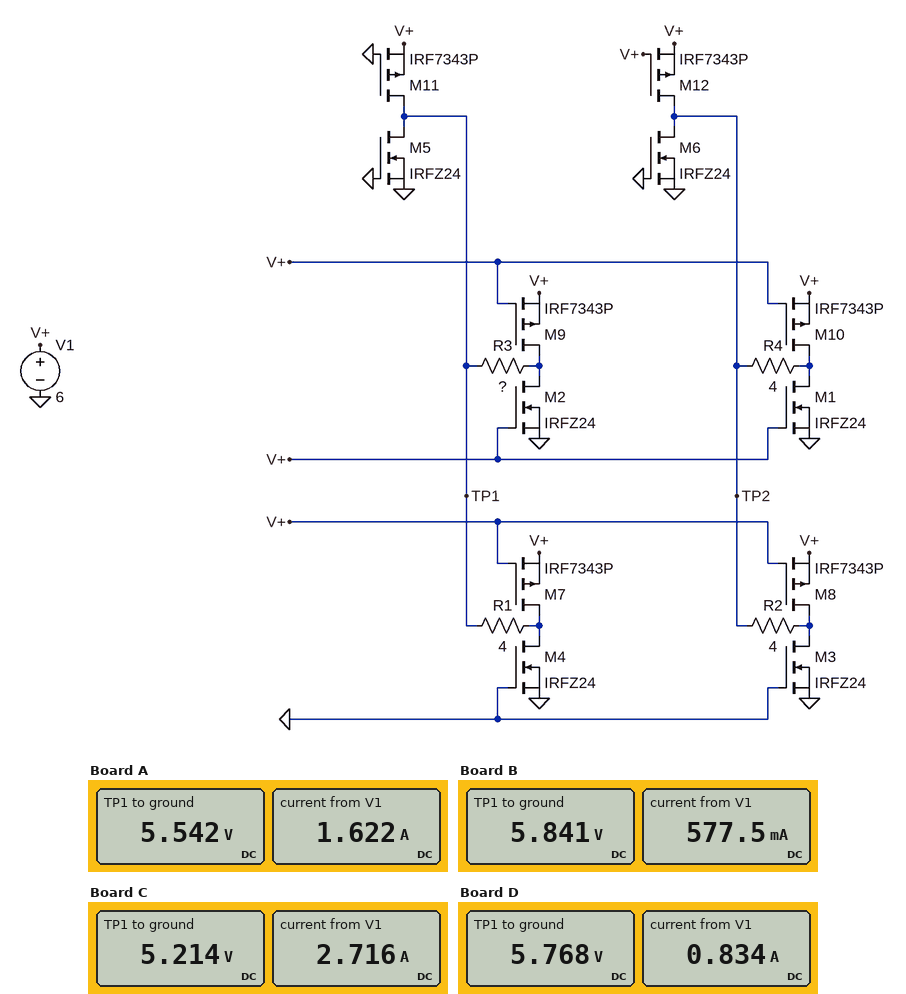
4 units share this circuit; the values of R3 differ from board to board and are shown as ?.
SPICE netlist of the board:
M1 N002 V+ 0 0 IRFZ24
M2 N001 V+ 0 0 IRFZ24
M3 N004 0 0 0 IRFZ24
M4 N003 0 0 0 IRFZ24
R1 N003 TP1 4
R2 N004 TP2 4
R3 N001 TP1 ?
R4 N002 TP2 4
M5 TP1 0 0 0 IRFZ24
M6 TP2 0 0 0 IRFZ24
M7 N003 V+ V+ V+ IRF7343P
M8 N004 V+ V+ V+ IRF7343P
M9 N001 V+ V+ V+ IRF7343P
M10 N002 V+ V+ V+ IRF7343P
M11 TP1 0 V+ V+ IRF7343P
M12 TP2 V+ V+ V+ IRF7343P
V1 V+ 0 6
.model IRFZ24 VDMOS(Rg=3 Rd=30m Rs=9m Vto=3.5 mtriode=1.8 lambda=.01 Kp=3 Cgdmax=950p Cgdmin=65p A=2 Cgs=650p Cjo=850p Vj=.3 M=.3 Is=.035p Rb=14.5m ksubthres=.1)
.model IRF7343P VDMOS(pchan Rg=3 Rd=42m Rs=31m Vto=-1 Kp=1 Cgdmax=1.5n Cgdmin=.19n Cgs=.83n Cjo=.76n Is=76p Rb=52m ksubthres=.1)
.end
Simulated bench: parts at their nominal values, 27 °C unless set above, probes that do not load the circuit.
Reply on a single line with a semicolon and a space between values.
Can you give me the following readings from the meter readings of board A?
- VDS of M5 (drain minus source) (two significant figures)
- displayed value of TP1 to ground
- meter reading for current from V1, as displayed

5.5 V; 5.542 V; 1.622 A
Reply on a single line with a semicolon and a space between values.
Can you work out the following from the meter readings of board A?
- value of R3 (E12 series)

3.3 Ω
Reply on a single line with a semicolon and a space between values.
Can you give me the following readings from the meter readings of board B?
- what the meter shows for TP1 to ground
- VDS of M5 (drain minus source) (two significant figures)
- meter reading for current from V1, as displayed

5.841 V; 5.8 V; 577.5 mA
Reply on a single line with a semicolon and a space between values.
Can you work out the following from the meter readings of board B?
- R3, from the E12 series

10 Ω
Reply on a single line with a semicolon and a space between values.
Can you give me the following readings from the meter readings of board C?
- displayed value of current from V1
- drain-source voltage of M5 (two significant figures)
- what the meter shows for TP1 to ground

2.716 A; 5.2 V; 5.214 V
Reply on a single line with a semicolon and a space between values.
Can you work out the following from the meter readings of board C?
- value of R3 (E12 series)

1.8 Ω
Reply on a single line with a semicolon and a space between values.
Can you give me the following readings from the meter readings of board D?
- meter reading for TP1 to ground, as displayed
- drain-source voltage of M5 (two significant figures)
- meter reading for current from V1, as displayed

5.768 V; 5.8 V; 0.834 A
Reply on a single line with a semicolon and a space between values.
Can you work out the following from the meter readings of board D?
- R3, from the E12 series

6.8 Ω
